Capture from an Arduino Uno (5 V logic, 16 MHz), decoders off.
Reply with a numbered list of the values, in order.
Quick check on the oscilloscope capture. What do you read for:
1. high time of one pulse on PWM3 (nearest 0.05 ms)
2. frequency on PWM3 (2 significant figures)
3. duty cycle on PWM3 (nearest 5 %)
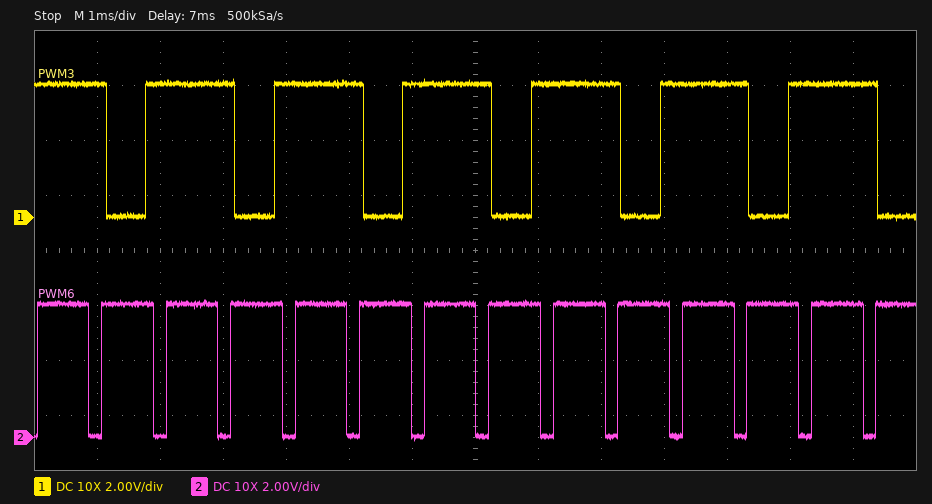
1. 1.40 ms
2. 490 Hz
3. 70 %
